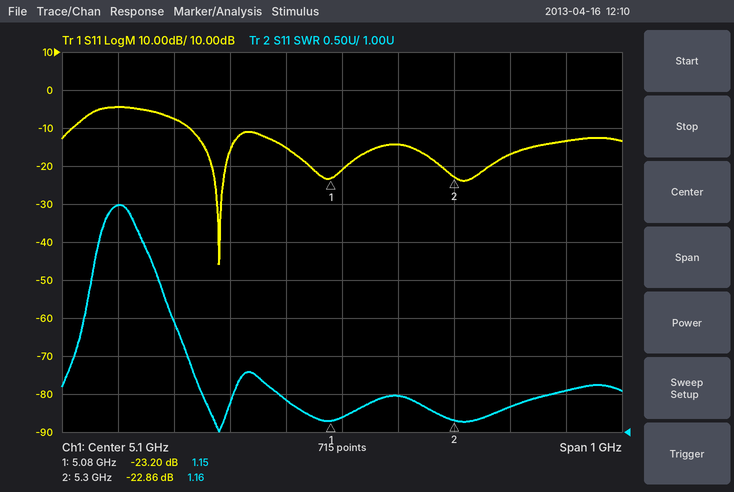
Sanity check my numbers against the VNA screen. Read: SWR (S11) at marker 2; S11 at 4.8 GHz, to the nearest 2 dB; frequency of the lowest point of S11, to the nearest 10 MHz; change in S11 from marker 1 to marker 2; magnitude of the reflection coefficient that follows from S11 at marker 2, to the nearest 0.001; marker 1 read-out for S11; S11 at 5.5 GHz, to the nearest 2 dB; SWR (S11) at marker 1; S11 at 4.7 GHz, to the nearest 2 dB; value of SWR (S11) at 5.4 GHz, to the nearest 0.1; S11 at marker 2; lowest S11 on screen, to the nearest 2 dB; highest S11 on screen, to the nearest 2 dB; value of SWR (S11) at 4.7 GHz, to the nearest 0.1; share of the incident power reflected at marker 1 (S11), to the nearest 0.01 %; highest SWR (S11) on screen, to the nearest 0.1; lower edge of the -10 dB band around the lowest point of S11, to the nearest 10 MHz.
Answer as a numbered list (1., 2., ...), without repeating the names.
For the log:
1. 1.16
2. -8 dB
3. 4.88 GHz
4. 0.34 dB
5. 0.072
6. -23.20 dB
7. -14 dB
8. 1.15
9. -4 dB
10. 1.3
11. -22.86 dB
12. -46 dB
13. -4 dB
14. 4.0
15. 0.48 %
16. 4.0
17. 4.83 GHz
